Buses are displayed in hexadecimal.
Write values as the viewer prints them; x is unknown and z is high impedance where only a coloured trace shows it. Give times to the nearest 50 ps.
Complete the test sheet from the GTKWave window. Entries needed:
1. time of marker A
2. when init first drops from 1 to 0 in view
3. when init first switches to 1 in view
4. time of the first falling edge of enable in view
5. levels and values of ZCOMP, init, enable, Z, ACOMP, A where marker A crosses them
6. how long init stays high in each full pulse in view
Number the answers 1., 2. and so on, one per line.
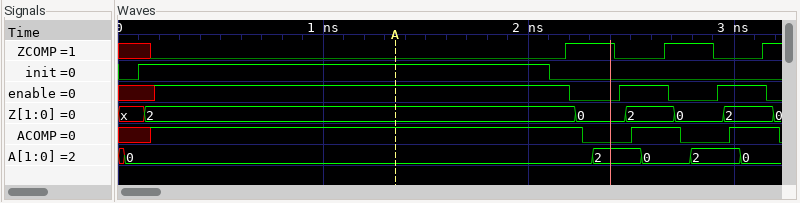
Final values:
1. 1350 ps
2. 2100 ps
3. 100 ps
4. 2200 ps
5. ZCOMP=0, init=1, enable=1, Z=2, ACOMP=1, A=0
6. 2000 ps
